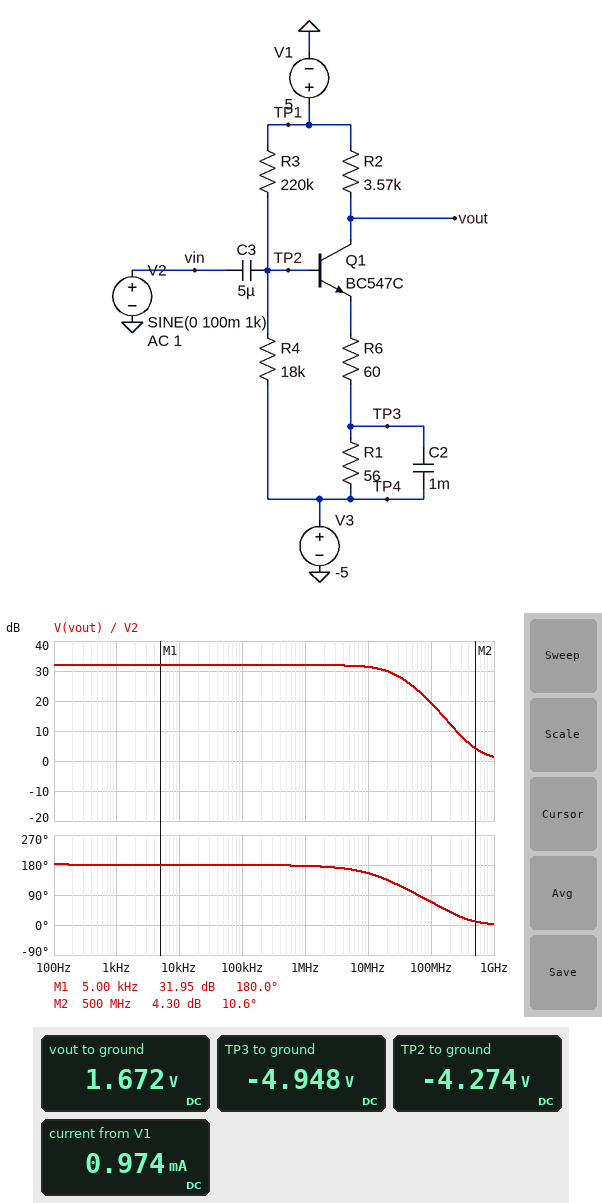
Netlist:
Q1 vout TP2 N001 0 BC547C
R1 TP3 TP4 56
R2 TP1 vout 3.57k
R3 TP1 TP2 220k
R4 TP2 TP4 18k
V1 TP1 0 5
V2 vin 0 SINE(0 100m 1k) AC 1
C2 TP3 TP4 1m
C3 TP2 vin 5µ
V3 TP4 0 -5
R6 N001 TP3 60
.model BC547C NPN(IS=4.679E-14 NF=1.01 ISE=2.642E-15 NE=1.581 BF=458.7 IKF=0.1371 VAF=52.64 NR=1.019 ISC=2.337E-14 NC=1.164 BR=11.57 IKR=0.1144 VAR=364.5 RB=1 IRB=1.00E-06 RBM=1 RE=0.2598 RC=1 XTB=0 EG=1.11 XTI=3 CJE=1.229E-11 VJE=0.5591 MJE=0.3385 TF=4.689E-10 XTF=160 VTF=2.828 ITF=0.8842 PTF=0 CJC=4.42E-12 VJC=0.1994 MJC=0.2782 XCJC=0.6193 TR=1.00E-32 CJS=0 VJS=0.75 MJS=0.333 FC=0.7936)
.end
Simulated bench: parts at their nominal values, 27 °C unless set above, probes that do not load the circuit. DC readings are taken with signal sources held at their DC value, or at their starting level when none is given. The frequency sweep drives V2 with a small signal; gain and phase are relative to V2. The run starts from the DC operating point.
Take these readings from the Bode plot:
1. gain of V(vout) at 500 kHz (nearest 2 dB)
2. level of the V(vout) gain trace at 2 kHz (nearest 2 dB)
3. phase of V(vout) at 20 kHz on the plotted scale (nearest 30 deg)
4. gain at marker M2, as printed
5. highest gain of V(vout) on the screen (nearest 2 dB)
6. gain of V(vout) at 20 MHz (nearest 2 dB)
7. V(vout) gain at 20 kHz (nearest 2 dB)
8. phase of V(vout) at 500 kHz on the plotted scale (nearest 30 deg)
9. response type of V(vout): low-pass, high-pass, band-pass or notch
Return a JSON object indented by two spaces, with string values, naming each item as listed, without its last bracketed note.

{
  "gain of V(vout) at 500 kHz": "32 dB",
  "level of the V(vout) gain trace at 2 kHz": "32 dB",
  "phase of V(vout) at 20 kHz on the plotted scale": "180 deg",
  "gain at marker M2, as printed": "4.30 dB",
  "highest gain of V(vout) on the screen": "32 dB",
  "gain of V(vout) at 20 MHz": "30 dB",
  "V(vout) gain at 20 kHz": "32 dB",
  "phase of V(vout) at 500 kHz on the plotted scale": "180 deg",
  "response type of V(vout): low-pass, high-pass, band-pass or notch": "low-pass"
}
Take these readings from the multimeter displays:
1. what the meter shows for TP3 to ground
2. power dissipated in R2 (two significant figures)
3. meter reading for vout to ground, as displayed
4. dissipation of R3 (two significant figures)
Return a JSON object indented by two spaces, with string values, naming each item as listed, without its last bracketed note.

{
  "what the meter shows for TP3 to ground": "-4.948 V",
  "power dissipated in R2": "3.1 mW",
  "meter reading for vout to ground, as displayed": "1.672 V",
  "dissipation of R3": "390 µW"
}
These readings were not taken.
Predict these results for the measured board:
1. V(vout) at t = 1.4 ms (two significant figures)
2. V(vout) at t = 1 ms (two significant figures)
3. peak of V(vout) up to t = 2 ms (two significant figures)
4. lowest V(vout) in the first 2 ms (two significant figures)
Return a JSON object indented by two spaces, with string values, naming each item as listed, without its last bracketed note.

{
  "V(vout) at t = 1.4 ms": "-810 mV",
  "V(vout) at t = 1 ms": "1.7 V",
  "peak of V(vout) up to t = 2 ms": "4.5 V",
  "lowest V(vout) in the first 2 ms": "-2.8 V"
}
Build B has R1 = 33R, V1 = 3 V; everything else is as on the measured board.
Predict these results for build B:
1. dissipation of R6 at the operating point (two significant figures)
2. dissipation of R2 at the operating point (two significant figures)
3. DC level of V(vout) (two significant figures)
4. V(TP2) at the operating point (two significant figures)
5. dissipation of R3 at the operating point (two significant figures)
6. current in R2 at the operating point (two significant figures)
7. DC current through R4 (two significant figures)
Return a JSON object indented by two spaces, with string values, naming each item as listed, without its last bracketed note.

{
  "dissipation of R6 at the operating point": "2.8 µW",
  "dissipation of R2 at the operating point": "160 µW",
  "DC level of V(vout)": "2.2 V",
  "V(TP2) at the operating point": "-4.4 V",
  "dissipation of R3 at the operating point": "250 µW",
  "current in R2 at the operating point": "210 µA",
  "DC current through R4": "33 µA"
}
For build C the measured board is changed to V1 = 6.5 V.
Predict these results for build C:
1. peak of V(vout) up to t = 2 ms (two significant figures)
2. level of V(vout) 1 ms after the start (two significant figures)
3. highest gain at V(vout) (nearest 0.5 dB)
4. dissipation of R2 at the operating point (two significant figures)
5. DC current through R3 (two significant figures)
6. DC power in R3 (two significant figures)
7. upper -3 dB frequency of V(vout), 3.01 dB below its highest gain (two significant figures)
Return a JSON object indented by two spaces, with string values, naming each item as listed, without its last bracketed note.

{
  "peak of V(vout) up to t = 2 ms": "4.8 V",
  "level of V(vout) 1 ms after the start": "840 mV",
  "highest gain at V(vout)": "33.0 dB",
  "dissipation of R2 at the operating point": "9.0 mW",
  "DC current through R3": "49 µA",
  "DC power in R3": "520 µW",
  "upper -3 dB frequency of V(vout), 3.01 dB below its highest gain": "25 MHz"
}
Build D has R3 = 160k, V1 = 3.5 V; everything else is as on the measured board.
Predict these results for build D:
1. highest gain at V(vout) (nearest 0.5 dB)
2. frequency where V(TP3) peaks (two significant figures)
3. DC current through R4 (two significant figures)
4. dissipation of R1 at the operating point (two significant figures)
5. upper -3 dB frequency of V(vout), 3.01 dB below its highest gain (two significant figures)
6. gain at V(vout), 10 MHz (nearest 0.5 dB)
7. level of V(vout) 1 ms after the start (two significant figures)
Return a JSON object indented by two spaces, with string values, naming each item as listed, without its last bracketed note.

{
  "highest gain at V(vout)": "33.0 dB",
  "frequency where V(TP3) peaks": "3.5 Hz",
  "DC current through R4": "45 µA",
  "dissipation of R1 at the operating point": "130 µW",
  "upper -3 dB frequency of V(vout), 3.01 dB below its highest gain": "20 MHz",
  "gain at V(vout), 10 MHz": "32.0 dB",
  "level of V(vout) 1 ms after the start": "-1.5 V"
}
